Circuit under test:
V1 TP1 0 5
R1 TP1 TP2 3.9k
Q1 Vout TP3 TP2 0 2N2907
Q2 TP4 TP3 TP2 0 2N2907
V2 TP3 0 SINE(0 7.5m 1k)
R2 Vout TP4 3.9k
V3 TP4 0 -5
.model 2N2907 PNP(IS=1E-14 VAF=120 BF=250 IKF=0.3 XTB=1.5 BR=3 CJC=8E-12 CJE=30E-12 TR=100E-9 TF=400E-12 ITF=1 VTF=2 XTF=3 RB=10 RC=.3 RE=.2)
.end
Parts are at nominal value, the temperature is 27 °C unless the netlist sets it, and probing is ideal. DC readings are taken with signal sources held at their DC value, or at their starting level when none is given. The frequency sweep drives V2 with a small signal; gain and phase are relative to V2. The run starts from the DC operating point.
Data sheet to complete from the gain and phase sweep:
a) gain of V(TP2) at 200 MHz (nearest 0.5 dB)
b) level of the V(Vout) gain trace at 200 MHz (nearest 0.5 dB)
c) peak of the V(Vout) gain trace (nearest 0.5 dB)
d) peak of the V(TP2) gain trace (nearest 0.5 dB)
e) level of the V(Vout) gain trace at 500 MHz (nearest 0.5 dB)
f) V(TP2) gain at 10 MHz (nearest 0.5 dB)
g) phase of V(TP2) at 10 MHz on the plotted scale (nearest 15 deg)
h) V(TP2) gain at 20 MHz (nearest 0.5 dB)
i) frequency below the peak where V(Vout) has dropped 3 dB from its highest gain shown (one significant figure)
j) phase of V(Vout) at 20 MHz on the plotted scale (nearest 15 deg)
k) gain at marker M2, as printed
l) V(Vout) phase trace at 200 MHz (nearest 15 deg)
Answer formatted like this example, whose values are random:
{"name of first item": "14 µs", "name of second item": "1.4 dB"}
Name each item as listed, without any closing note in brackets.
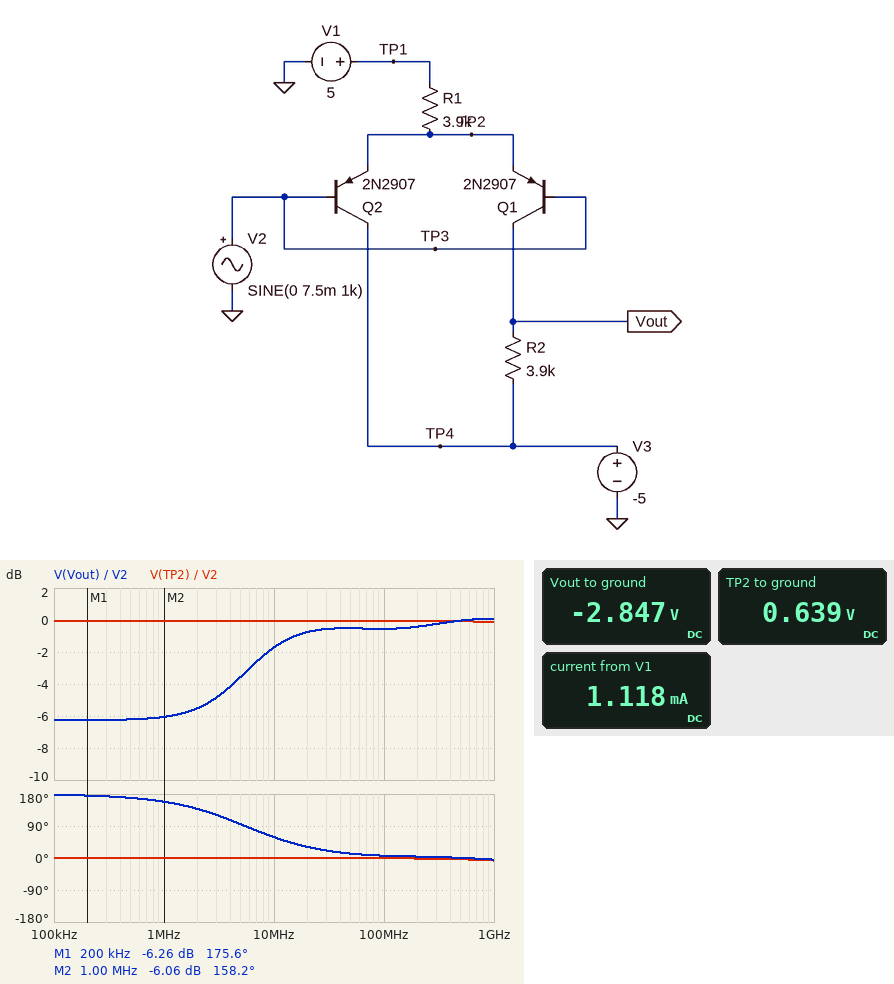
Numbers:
{"gain of V(TP2) at 200 MHz": "0 dB", "level of the V(Vout) gain trace at 200 MHz": "-0.5 dB", "peak of the V(Vout) gain trace": "0 dB", "peak of the V(TP2) gain trace": "0 dB", "level of the V(Vout) gain trace at 500 MHz": "0 dB", "V(TP2) gain at 10 MHz": "0 dB", "phase of V(TP2) at 10 MHz on the plotted scale": "0 deg", "V(TP2) gain at 20 MHz": "0 dB", "frequency below the peak where V(Vout) has dropped 3 dB from its highest gain shown": "6 MHz", "phase of V(Vout) at 20 MHz on the plotted scale": "30 deg", "gain at marker M2, as printed": "-6.06 dB", "V(Vout) phase trace at 200 MHz": "0 deg"}
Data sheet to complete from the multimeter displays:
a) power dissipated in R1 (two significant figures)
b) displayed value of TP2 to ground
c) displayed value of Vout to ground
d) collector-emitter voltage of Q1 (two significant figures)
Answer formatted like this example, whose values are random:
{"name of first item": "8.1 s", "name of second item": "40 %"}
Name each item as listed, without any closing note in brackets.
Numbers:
{"power dissipated in R1": "4.9 mW", "displayed value of TP2 to ground": "0.639 V", "displayed value of Vout to ground": "-2.847 V", "collector-emitter voltage of Q1": "-3.5 V"}
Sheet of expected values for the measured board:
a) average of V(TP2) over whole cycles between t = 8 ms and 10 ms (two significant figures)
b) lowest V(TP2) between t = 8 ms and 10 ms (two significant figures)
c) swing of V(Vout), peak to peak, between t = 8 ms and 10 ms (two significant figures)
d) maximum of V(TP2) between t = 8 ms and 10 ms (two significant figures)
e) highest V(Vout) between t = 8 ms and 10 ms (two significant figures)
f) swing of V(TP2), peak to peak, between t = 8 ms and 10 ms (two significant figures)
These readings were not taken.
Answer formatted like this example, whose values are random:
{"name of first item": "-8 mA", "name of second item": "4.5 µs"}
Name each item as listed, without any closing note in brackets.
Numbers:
{"average of V(TP2) over whole cycles between t = 8 ms and 10 ms": "640 mV", "lowest V(TP2) between t = 8 ms and 10 ms": "630 mV", "swing of V(Vout), peak to peak, between t = 8 ms and 10 ms": "7.3 mV", "maximum of V(TP2) between t = 8 ms and 10 ms": "650 mV", "highest V(Vout) between t = 8 ms and 10 ms": "-2.8 V", "swing of V(TP2), peak to peak, between t = 8 ms and 10 ms": "15 mV"}
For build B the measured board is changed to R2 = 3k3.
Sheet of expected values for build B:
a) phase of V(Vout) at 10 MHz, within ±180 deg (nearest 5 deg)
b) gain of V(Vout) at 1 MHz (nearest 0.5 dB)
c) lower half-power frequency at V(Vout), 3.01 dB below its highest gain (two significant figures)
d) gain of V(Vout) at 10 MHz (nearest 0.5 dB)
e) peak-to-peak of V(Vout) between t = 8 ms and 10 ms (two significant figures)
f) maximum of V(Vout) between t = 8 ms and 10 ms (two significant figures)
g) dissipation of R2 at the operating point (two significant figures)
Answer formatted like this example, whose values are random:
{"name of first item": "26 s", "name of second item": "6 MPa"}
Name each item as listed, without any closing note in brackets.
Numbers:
{"phase of V(Vout) at 10 MHz, within ±180 deg": "65 deg", "gain of V(Vout) at 1 MHz": "-7.5 dB", "lower half-power frequency at V(Vout), 3.01 dB below its highest gain": "8.4 MHz", "gain of V(Vout) at 10 MHz": "-2.5 dB", "peak-to-peak of V(Vout) between t = 8 ms and 10 ms": "6.2 mV", "maximum of V(Vout) between t = 8 ms and 10 ms": "-3.2 V", "dissipation of R2 at the operating point": "1.0 mW"}
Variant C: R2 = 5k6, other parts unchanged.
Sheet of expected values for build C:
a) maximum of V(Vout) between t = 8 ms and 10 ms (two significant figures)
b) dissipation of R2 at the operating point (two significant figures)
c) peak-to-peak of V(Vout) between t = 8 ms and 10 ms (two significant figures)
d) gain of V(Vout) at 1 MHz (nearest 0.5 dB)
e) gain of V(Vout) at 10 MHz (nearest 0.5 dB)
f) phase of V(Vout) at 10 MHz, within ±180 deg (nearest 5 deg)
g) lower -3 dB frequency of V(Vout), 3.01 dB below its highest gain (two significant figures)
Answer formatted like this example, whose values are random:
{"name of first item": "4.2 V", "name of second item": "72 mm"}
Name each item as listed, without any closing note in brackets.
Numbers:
{"maximum of V(Vout) between t = 8 ms and 10 ms": "-1.9 V", "dissipation of R2 at the operating point": "1.7 mW", "peak-to-peak of V(Vout) between t = 8 ms and 10 ms": "10 mV", "gain of V(Vout) at 1 MHz": "-3.0 dB", "gain of V(Vout) at 10 MHz": "-0.5 dB", "phase of V(Vout) at 10 MHz, within ±180 deg": "45 deg", "lower -3 dB frequency of V(Vout), 3.01 dB below its highest gain": "1.3 MHz"}
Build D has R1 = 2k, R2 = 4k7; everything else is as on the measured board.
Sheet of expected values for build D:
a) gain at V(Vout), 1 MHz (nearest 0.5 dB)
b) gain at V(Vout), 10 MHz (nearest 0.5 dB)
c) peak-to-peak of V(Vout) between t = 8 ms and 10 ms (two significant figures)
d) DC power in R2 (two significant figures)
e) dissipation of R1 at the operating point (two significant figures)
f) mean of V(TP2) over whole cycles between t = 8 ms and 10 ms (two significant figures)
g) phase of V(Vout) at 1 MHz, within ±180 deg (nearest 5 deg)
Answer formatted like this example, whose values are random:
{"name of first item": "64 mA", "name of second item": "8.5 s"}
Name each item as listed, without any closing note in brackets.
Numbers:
{"gain at V(Vout), 1 MHz": "1.0 dB", "gain at V(Vout), 10 MHz": "-0.5 dB", "peak-to-peak of V(Vout) between t = 8 ms and 10 ms": "17 mV", "DC power in R2": "5.3 mW", "dissipation of R1 at the operating point": "9.4 mW", "mean of V(TP2) over whole cycles between t = 8 ms and 10 ms": "660 mV", "phase of V(Vout) at 1 MHz, within ±180 deg": "150 deg"}
